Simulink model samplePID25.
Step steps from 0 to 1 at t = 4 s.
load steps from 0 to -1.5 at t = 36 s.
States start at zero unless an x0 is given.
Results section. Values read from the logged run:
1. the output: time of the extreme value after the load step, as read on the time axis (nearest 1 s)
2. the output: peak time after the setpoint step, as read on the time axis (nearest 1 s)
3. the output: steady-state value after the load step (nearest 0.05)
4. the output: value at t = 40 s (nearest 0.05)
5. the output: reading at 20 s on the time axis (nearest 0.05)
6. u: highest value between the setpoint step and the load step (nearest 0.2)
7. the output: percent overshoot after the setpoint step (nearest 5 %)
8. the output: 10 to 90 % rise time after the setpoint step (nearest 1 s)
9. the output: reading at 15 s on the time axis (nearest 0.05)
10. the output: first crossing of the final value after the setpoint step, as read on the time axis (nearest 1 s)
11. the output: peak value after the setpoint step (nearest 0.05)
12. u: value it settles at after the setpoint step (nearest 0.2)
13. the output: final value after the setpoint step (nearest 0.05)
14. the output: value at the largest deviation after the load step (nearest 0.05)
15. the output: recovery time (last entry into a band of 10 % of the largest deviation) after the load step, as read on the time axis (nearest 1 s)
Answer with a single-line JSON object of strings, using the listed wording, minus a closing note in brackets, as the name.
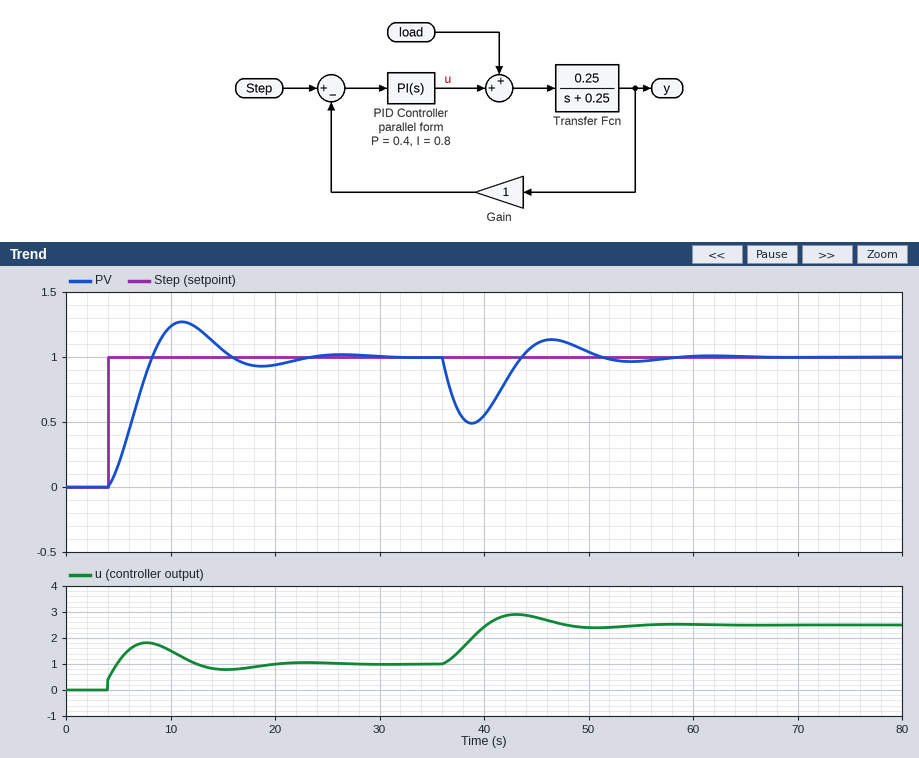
{"the output: time of the extreme value after the load step, as read on the time axis": "39 s", "the output: peak time after the setpoint step, as read on the time axis": "11 s", "the output: steady-state value after the load step": "1.00", "the output: value at t = 40 s": "0.55", "the output: reading at 20 s on the time axis": "0.95", "u: highest value between the setpoint step and the load step": "1.8", "the output: percent overshoot after the setpoint step": "25 %", "the output: 10 to 90 % rise time after the setpoint step": "3 s", "the output: reading at 15 s on the time axis": "1.05", "the output: first crossing of the final value after the setpoint step, as read on the time axis": "8 s", "the output: peak value after the setpoint step": "1.25", "u: value it settles at after the setpoint step": "1.0", "the output: final value after the setpoint step": "1.00", "the output: value at the largest deviation after the load step": "0.50", "the output: recovery time (last entry into a band of 10 % of the largest deviation) after the load step, as read on the time axis": "50 s"}
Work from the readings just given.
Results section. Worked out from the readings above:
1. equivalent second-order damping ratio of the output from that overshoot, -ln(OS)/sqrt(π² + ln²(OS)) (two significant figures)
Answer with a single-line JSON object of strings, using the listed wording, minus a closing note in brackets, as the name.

{"equivalent second-order damping ratio of the output from that overshoot, -ln(OS)/sqrt(π² + ln²(OS))": "0.40"}
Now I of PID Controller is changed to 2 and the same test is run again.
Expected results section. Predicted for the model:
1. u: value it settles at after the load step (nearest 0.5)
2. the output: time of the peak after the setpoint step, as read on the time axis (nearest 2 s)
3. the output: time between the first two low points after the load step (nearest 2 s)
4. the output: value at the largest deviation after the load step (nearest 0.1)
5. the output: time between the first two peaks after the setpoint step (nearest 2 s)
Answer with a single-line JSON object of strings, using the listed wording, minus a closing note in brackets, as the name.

{"u: value it settles at after the load step": "2.5", "the output: time of the peak after the setpoint step, as read on the time axis": "8 s", "the output: time between the first two low points after the load step": "10 s", "the output: value at the largest deviation after the load step": "0.6", "the output: time between the first two peaks after the setpoint step": "10 s"}
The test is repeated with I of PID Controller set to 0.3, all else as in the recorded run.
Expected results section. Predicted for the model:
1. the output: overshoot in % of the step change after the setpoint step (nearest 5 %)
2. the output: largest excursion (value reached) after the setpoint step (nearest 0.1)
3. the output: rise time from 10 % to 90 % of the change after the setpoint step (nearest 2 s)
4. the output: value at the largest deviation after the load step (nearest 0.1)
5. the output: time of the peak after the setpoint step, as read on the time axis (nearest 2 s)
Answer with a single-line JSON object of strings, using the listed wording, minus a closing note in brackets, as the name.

{"the output: overshoot in % of the step change after the setpoint step": "10 %", "the output: largest excursion (value reached) after the setpoint step": "1.1", "the output: rise time from 10 % to 90 % of the change after the setpoint step": "6 s", "the output: value at the largest deviation after the load step": "0.3", "the output: time of the peak after the setpoint step, as read on the time axis": "18 s"}
